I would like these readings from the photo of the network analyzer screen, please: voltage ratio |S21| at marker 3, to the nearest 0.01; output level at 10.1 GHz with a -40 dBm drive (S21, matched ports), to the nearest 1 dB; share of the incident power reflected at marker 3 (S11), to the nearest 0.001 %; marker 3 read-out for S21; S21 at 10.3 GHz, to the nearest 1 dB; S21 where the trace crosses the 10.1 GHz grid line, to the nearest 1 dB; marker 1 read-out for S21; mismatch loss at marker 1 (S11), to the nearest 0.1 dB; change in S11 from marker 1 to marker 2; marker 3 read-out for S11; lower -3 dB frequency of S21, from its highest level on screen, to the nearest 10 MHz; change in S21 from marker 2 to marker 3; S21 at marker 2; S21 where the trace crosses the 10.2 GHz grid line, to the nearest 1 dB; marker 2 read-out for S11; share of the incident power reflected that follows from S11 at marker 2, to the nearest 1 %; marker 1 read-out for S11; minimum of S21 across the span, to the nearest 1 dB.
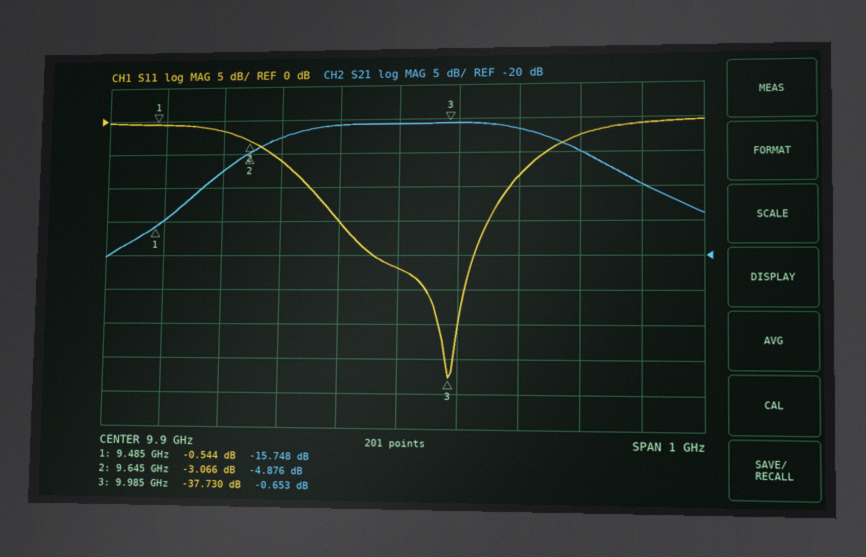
0.93
-42 dBm
0.017 %
-0.653 dB
-10 dB
-2 dB
-15.748 dB
9.3 dB
-2.522 dB
-37.730 dB
9.67 GHz
4.223 dB
-4.876 dB
-5 dB
-3.066 dB
49 %
-0.544 dB
-20 dB
